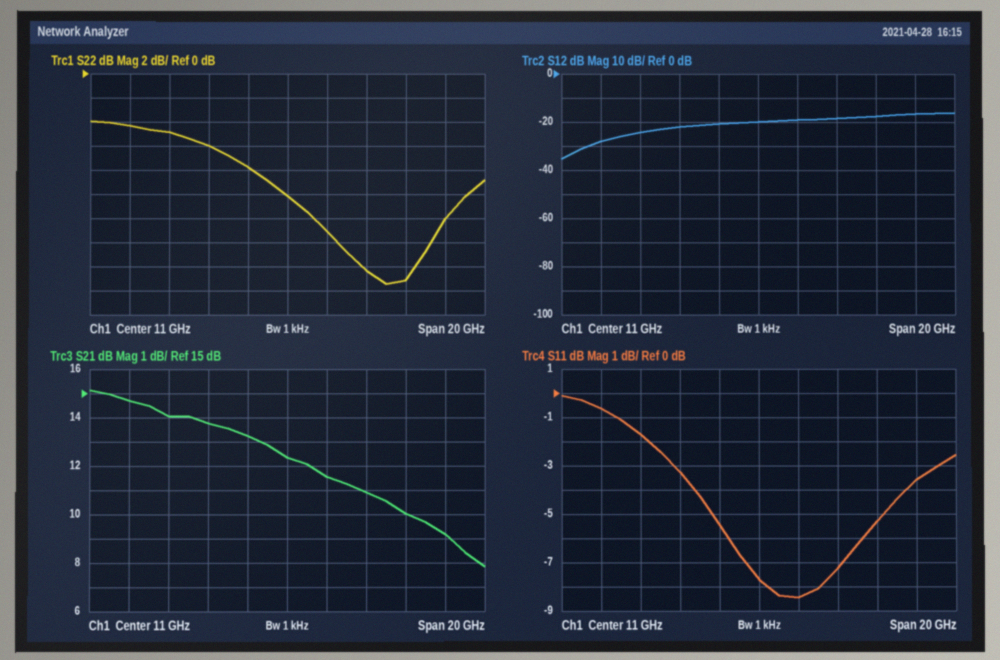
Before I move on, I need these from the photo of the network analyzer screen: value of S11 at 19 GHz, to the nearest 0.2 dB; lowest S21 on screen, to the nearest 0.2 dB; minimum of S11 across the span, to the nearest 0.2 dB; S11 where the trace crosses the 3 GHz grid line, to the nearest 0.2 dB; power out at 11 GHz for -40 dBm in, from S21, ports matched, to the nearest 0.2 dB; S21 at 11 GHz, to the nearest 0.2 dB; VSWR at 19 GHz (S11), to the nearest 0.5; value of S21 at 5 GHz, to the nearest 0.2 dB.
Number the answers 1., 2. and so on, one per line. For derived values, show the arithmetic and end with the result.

1. -3.6 dB
2. 7.8 dB
3. -8.4 dB
4. -0.6 dB
5. -40 dBm + (12.4 dB) = -27.6 dBm
6. 12.4 dB
7. |Γ| = 10^(-3.6/20) = 0.6607; VSWR = (1 + 0.6607)/(1 − 0.6607) ≈ 4.89, so 5.0 to the nearest 0.5
8. 14.0 dB
